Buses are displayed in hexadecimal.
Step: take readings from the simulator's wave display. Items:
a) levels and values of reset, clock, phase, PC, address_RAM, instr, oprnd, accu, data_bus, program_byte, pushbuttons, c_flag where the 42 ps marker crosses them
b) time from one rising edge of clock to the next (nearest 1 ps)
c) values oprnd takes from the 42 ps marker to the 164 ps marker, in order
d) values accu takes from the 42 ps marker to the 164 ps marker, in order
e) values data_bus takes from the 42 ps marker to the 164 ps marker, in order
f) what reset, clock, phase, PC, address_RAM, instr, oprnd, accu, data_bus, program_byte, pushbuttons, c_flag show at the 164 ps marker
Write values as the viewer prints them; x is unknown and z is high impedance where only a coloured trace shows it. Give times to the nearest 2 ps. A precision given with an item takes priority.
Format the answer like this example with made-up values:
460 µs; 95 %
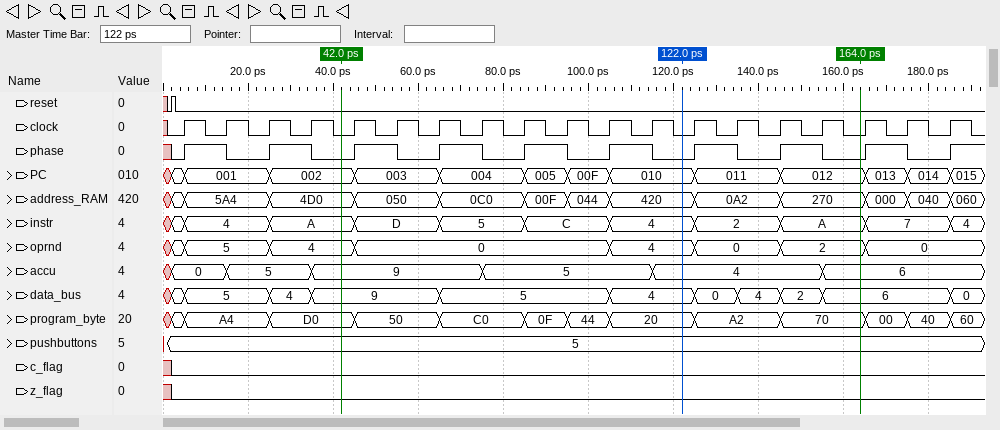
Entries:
reset=0, clock=0, phase=0, PC=002, address_RAM=4D0, instr=A, oprnd=4, accu=9, data_bus=9, program_byte=D0, pushbuttons=5, c_flag=0; 10 ps; 4, 0, 4, 0, 2; 9, 5, 4, 6; 9, 5, 4, 0, 4, 2, 6; reset=0, clock=0, phase=0, PC=012, address_RAM=270, instr=A, oprnd=2, accu=6, data_bus=6, program_byte=70, pushbuttons=5, c_flag=0
